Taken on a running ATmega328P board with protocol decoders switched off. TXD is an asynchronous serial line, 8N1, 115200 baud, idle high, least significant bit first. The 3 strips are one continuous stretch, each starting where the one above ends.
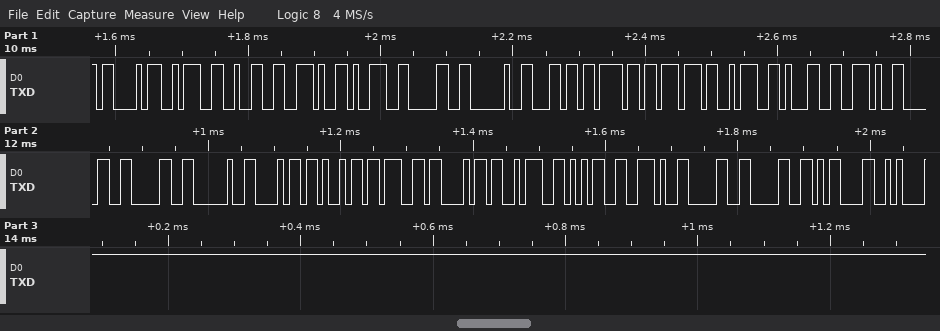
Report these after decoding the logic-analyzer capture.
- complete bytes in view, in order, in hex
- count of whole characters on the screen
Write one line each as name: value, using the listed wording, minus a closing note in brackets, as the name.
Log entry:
complete bytes in view, in order, in hex: 43 3A 32 2E 39 30 20 6C 6F 77 3A 31 2E 30 30 20 68 69 67 68 3A 35 2E 30 30 0D 0A
count of whole characters on the screen: 27
